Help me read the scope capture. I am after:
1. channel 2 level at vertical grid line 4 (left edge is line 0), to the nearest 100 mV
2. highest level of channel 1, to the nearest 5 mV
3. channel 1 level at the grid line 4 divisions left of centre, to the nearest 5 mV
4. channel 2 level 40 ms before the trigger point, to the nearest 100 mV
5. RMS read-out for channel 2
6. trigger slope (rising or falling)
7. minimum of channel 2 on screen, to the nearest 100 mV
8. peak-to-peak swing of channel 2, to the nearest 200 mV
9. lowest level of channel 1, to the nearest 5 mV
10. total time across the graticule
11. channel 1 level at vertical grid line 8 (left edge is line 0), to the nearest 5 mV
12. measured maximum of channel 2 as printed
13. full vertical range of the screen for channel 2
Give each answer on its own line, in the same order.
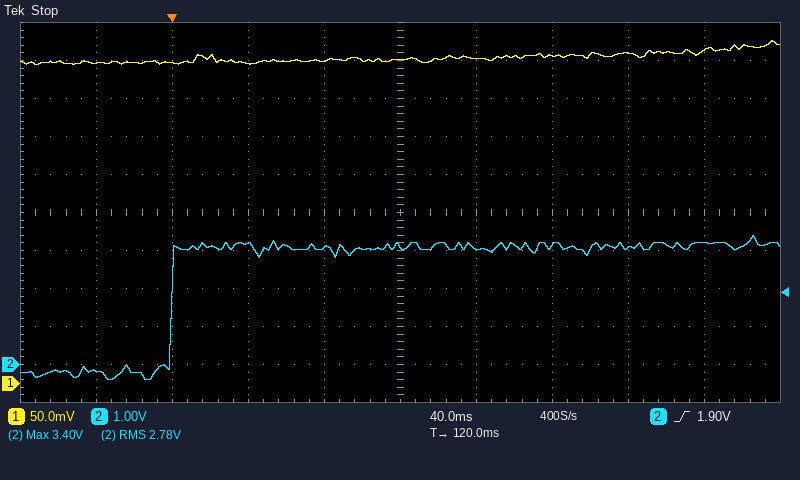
3.1 V
450 mV
420 mV
-200 mV
2.78 V
rising
-400 mV
3.8 V
420 mV
400 ms
435 mV
3.40 V
10 V
